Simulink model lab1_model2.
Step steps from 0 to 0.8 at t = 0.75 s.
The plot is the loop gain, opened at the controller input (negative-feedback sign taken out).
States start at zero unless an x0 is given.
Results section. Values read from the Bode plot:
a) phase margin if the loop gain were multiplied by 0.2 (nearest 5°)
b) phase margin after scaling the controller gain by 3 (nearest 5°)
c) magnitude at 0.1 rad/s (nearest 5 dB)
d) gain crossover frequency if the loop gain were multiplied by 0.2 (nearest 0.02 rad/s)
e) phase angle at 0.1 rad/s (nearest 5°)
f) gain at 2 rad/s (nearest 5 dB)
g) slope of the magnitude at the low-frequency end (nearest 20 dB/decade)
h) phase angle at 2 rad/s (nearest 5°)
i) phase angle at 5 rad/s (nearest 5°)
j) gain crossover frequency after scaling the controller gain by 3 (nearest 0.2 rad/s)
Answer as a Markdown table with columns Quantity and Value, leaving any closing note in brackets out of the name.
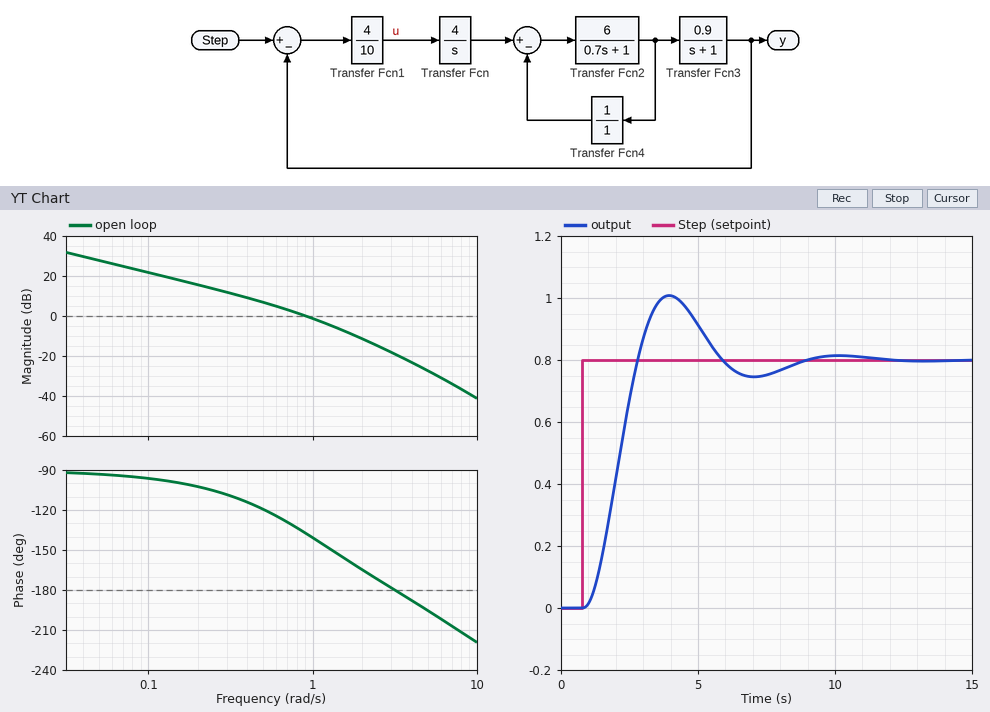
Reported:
| Quantity | Value |
|---|---|
| phase margin if the loop gain were multiplied by 0.2 | 75° |
| phase margin after scaling the controller gain by 3 | 20° |
| magnitude at 0.1 rad/s | 20 dB |
| gain crossover frequency if the loop gain were multiplied by 0.2 | 0.24 rad/s |
| phase angle at 0.1 rad/s | -95° |
| gain at 2 rad/s | -10 dB |
| slope of the magnitude at the low-frequency end | -20 dB/decade |
| phase angle at 2 rad/s | -165° |
| phase angle at 5 rad/s | -195° |
| gain crossover frequency after scaling the controller gain by 3 | 1.8 rad/s |
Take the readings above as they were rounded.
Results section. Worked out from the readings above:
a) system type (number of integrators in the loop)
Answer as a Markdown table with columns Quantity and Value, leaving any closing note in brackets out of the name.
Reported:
| Quantity | Value |
|---|---|
| system type | 1 |
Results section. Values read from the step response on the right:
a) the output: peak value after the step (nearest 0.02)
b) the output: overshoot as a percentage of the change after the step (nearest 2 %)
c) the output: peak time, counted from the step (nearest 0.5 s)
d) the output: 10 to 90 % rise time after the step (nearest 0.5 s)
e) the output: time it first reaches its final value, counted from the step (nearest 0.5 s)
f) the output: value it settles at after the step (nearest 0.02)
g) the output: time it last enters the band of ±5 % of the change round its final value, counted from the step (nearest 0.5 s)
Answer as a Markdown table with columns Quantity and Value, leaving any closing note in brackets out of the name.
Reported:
| Quantity | Value |
|---|---|
| the output: peak value after the step | 1.00 |
| the output: overshoot as a percentage of the change after the step | 26 % |
| the output: peak time, counted from the step | 3.0 s |
| the output: 10 to 90 % rise time after the step | 1.5 s |
| the output: time it first reaches its final value, counted from the step | 2.0 s |
| the output: value it settles at after the step | 0.80 |
| the output: time it last enters the band of ±5 % of the change round its final value, counted from the step | 7.0 s |
